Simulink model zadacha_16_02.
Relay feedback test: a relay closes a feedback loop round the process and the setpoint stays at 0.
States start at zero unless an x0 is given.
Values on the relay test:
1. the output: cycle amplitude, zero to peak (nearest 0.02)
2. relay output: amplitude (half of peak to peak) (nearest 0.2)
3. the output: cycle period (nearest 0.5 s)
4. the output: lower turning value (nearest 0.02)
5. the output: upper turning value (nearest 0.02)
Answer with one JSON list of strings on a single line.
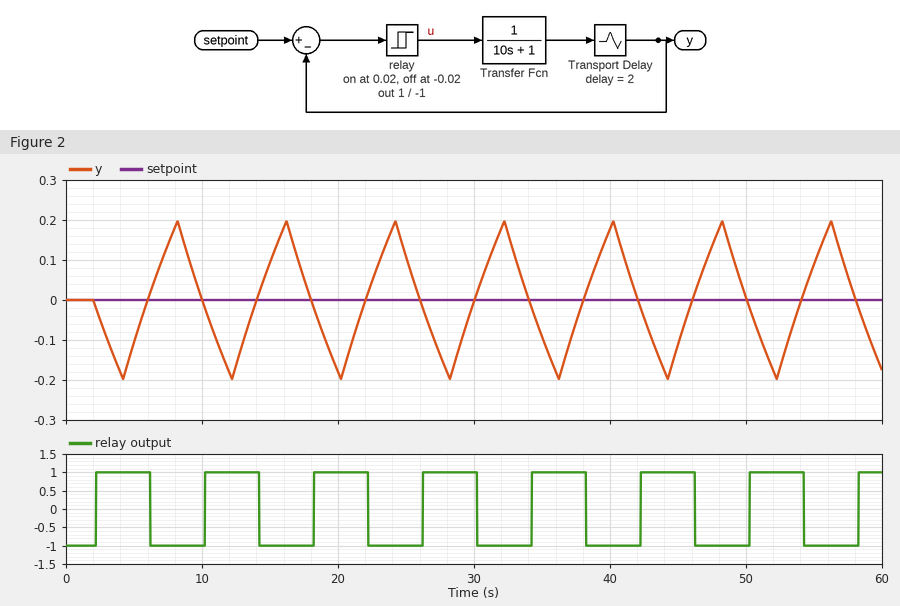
["0.20", "1.0", "8.0 s", "-0.20", "0.20"]
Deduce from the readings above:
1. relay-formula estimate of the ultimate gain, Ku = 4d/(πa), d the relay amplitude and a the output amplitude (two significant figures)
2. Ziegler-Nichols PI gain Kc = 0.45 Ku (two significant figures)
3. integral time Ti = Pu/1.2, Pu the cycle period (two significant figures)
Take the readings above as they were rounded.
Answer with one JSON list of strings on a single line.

["6.4", "2.9", "6.7 s"]
